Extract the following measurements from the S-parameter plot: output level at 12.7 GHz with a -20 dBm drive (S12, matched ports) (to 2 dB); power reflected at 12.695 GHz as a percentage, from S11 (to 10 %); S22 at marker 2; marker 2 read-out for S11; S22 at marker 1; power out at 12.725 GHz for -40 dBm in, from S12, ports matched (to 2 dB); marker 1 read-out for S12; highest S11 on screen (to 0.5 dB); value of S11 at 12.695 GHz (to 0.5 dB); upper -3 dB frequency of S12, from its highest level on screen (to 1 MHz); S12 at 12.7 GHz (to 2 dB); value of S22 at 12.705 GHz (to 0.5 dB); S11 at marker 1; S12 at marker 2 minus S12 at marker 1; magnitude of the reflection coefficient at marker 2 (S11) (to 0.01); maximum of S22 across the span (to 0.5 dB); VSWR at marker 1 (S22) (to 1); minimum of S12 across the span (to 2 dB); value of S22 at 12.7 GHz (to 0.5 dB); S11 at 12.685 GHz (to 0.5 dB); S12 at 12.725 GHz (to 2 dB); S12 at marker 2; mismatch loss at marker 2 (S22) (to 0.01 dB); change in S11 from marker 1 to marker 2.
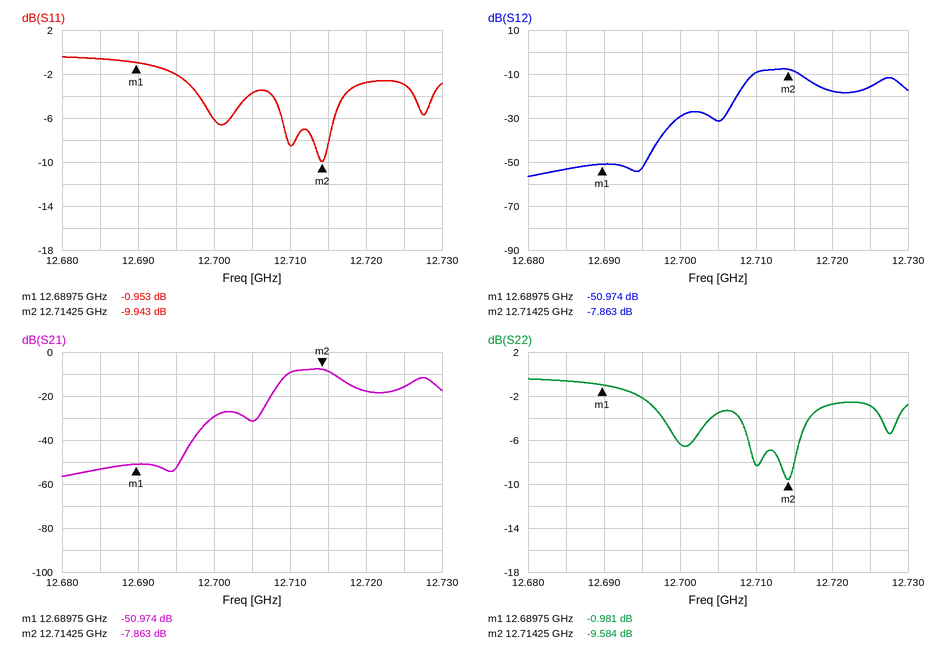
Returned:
-50 dBm
60 %
-9.584 dB
-9.943 dB
-0.981 dB
-56 dBm
-50.974 dB
-0.5 dB
-2.0 dB
12.716 GHz
-30 dB
-3.5 dB
-0.953 dB
43.111 dB
0.32
-0.5 dB
18
-56 dB
-6.5 dB
-0.5 dB
-16 dB
-7.863 dB
0.51 dB
-8.990 dB
